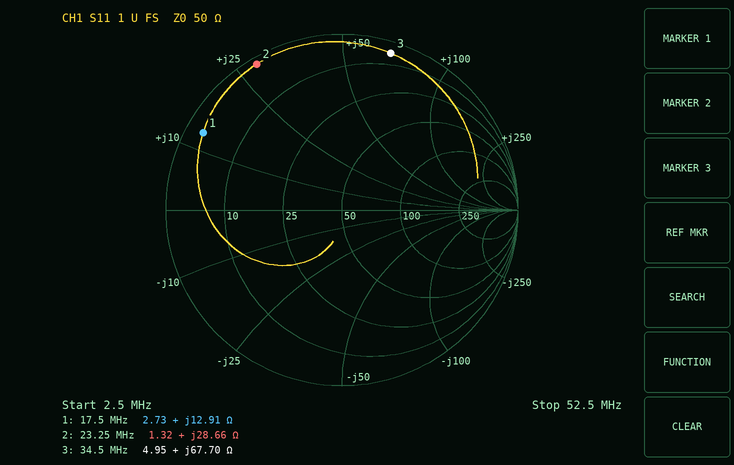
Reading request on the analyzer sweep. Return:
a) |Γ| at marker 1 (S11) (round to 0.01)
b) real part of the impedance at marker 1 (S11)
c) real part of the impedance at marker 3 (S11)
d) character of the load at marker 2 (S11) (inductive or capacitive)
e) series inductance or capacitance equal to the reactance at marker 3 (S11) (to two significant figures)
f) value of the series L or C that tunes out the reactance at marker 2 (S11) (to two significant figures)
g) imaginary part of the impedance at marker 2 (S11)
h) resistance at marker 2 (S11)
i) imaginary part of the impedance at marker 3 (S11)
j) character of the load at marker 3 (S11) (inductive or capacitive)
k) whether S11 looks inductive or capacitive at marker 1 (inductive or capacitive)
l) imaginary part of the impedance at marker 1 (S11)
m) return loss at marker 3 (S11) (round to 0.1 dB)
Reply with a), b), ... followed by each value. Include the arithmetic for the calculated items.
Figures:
a) 0.90
b) 2.73 Ω
c) 4.95 Ω
d) inductive
e) L = 67.7 Ω/(2π × 34.5 MHz) ≈ 312 nH, so 310 nH to two significant figures
f) C = 1/(2π × 23.25 MHz × 28.66 Ω) ≈ 239 pF, so 240 pF to two significant figures
g) +28.66 Ω
h) 1.32 Ω
i) +67.70 Ω
j) inductive
k) inductive
l) +12.91 Ω
m) 0.6 dB
